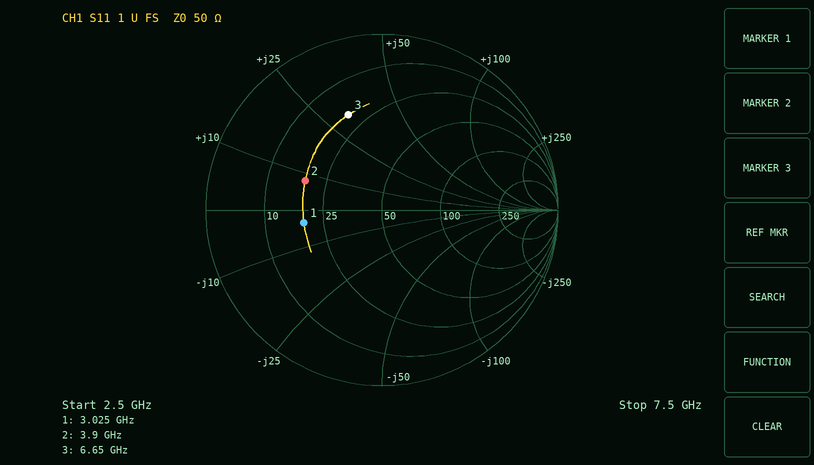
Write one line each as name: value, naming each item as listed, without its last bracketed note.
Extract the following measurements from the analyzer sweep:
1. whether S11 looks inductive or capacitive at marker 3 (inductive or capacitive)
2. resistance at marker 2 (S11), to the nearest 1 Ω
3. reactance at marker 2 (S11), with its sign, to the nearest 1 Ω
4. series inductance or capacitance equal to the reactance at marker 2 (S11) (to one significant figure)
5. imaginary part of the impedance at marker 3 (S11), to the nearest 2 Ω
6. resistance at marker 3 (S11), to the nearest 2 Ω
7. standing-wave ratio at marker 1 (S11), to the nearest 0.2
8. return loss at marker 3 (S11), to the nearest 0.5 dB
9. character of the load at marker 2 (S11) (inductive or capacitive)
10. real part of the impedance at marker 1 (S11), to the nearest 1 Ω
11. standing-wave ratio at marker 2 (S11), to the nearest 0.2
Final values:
whether S11 looks inductive or capacitive at marker 3: inductive
resistance at marker 2 (S11), to the nearest 1 Ω: 19 Ω
reactance at marker 2 (S11), with its sign, to the nearest 1 Ω: +8 Ω
series inductance or capacitance equal to the reactance at marker 2 (S11): 300 pH
imaginary part of the impedance at marker 3 (S11), to the nearest 2 Ω: +32 Ω
resistance at marker 3 (S11), to the nearest 2 Ω: 20 Ω
standing-wave ratio at marker 1 (S11), to the nearest 0.2: 2.6
return loss at marker 3 (S11), to the nearest 0.5 dB: 5.0 dB
character of the load at marker 2 (S11): inductive
real part of the impedance at marker 1 (S11), to the nearest 1 Ω: 19 Ω
standing-wave ratio at marker 2 (S11), to the nearest 0.2: 2.8
